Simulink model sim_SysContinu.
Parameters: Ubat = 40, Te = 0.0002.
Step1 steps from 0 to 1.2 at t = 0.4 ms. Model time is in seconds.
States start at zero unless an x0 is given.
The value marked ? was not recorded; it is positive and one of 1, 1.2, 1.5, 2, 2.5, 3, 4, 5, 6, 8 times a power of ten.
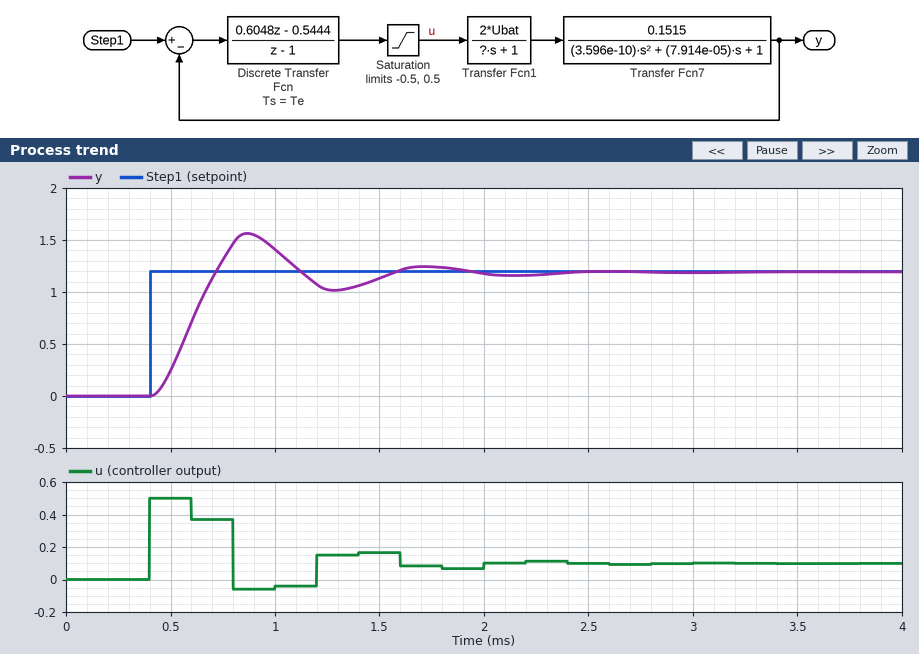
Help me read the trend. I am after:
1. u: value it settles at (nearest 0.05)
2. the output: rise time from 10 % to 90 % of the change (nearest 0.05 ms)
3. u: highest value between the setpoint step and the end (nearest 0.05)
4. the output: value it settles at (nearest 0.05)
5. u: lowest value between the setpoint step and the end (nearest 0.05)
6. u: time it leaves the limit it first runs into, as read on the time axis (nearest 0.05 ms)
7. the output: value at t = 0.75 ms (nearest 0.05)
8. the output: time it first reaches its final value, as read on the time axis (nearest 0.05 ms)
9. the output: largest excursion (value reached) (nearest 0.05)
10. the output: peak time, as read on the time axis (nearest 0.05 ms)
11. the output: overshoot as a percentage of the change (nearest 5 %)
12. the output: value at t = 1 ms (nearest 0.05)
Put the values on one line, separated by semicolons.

0.10; 0.20 ms; 0.50; 1.20; -0.05; 0.60 ms; 1.30; 0.70 ms; 1.55; 0.85 ms; 30 %; 1.40
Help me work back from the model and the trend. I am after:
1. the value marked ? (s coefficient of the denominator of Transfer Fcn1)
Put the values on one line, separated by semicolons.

0.001
